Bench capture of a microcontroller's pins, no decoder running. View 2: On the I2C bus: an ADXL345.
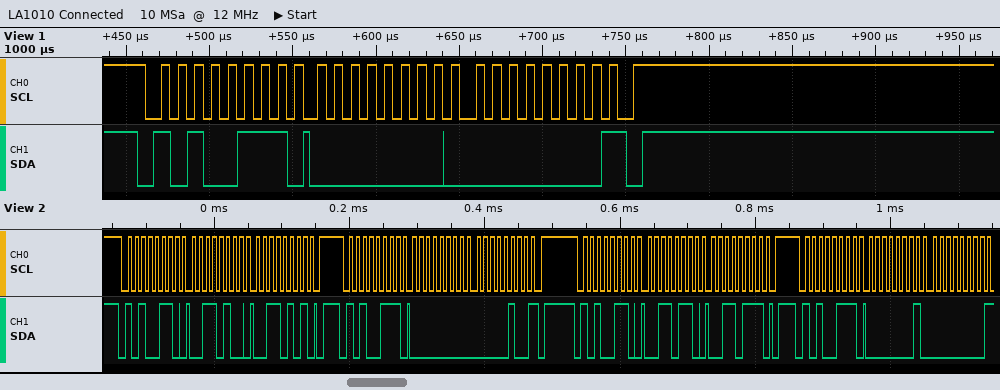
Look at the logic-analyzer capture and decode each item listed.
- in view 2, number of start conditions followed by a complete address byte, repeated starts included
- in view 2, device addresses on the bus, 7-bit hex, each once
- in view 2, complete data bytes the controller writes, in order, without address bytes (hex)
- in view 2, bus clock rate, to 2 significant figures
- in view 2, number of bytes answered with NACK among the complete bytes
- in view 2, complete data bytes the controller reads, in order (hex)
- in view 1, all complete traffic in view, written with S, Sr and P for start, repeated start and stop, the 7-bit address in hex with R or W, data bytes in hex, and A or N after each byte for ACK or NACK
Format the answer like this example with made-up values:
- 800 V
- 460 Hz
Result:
- 4
- 0x53
- 34 35 36 37
- 100 kHz
- 2
- 00 04 01 00
- S 53R A 00 A 00 N P
